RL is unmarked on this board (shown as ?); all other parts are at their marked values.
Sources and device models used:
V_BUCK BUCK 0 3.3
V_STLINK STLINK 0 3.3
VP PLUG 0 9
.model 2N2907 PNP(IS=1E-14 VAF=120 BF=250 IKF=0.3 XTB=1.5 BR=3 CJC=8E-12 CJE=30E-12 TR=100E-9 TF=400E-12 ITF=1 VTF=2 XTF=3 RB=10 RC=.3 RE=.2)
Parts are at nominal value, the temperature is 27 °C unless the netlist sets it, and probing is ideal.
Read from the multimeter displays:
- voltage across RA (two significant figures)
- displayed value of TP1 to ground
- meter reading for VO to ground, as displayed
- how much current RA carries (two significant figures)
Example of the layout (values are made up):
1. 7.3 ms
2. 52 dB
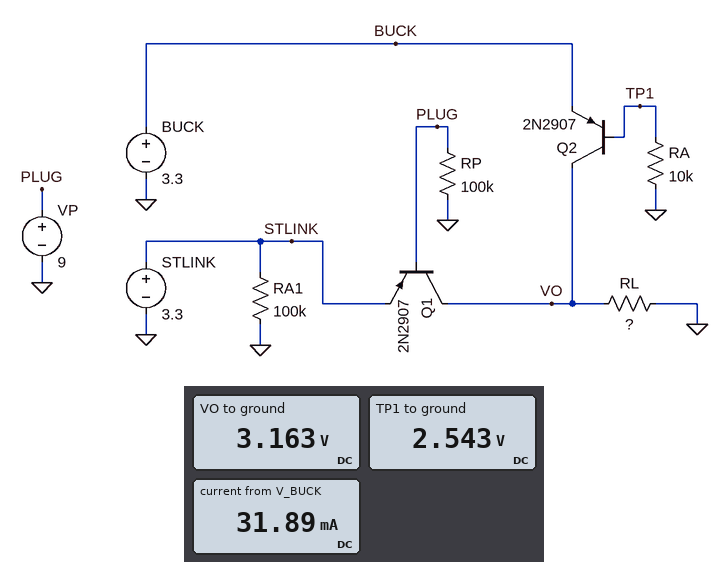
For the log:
1. 2.5 V
2. 2.543 V
3. 3.163 V
4. 250 µA
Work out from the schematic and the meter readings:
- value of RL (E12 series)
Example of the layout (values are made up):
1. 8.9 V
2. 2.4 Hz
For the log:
1. 100 Ω
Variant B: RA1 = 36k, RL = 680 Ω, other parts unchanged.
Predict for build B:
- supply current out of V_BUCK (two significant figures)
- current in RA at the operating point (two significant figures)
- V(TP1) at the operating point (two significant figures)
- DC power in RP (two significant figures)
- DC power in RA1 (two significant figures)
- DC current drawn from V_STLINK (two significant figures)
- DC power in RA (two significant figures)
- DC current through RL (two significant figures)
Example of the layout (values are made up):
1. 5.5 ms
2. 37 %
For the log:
1. 5.0 mA
2. 260 µA
3. 2.6 V
4. 810 µW
5. 300 µW
6. 92 µA
7. 670 µW
8. 4.8 mA
